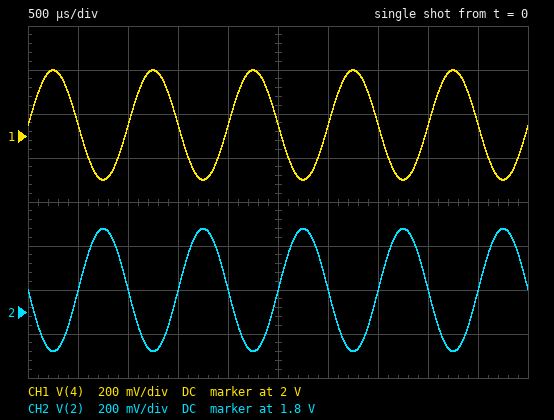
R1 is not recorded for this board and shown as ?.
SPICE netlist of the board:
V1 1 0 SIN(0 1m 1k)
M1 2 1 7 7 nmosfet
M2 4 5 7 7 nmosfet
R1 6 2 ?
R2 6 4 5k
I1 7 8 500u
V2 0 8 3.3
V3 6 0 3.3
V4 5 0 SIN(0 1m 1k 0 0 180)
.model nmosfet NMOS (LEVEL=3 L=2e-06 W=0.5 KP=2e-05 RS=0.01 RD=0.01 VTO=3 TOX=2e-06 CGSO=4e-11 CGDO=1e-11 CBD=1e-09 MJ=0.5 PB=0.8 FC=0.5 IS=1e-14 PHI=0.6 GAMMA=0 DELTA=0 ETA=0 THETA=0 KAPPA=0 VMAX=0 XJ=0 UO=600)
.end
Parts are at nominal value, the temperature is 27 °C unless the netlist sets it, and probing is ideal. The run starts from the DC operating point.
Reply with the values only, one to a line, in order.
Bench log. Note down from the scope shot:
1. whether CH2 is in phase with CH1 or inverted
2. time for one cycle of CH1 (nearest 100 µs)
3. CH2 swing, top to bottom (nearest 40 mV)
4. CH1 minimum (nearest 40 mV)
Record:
inverted
1.0 ms
560 mV
1.80 V
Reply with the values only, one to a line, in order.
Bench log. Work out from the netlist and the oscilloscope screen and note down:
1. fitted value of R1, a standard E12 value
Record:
5.6 kΩ
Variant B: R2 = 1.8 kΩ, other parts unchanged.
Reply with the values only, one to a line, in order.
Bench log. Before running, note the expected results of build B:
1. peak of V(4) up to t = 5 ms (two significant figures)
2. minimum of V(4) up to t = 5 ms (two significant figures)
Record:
2.9 V
2.8 V
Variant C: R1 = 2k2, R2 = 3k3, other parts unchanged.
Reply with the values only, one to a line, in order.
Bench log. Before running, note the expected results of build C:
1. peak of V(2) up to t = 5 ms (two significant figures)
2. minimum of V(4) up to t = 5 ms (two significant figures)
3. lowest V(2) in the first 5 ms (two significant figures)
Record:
2.9 V
2.3 V
2.6 V
